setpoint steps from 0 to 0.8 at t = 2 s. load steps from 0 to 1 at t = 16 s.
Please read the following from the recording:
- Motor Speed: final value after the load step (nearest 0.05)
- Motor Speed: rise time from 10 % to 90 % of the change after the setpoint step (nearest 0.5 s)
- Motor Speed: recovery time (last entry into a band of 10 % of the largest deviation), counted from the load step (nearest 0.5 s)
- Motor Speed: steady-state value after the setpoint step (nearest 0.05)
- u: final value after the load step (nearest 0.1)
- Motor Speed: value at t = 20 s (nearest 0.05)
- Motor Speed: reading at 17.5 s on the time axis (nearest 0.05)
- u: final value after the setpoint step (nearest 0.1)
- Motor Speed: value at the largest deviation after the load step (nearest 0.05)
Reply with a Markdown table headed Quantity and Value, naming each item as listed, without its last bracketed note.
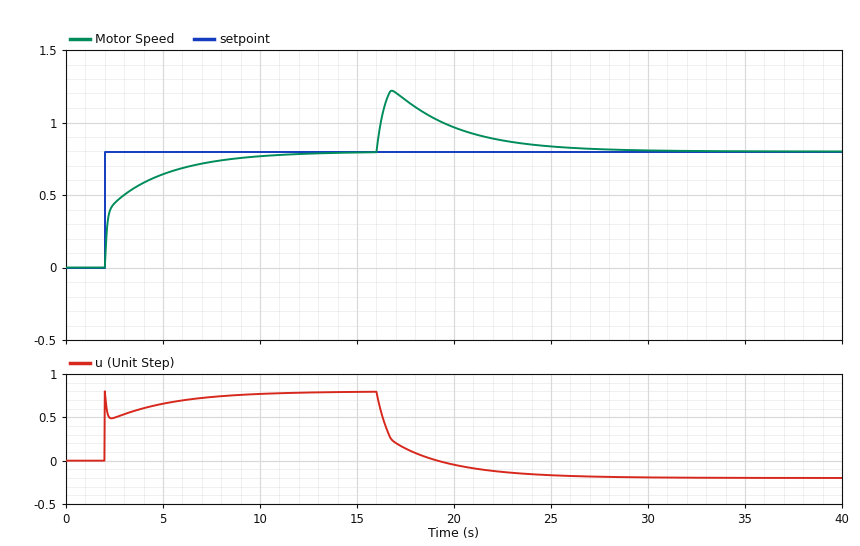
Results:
| Quantity | Value |
|---|---|
| Motor Speed: final value after the load step | 0.80 |
| Motor Speed: rise time from 10 % to 90 % of the change after the setpoint step | 5.0 s |
| Motor Speed: recovery time (last entry into a band of 10 % of the largest deviation), counted from the load step | 8.5 s |
| Motor Speed: steady-state value after the setpoint step | 0.80 |
| u: final value after the load step | -0.2 |
| Motor Speed: value at t = 20 s | 0.95 |
| Motor Speed: reading at 17.5 s on the time axis | 1.15 |
| u: final value after the setpoint step | 0.8 |
| Motor Speed: value at the largest deviation after the load step | 1.20 |
